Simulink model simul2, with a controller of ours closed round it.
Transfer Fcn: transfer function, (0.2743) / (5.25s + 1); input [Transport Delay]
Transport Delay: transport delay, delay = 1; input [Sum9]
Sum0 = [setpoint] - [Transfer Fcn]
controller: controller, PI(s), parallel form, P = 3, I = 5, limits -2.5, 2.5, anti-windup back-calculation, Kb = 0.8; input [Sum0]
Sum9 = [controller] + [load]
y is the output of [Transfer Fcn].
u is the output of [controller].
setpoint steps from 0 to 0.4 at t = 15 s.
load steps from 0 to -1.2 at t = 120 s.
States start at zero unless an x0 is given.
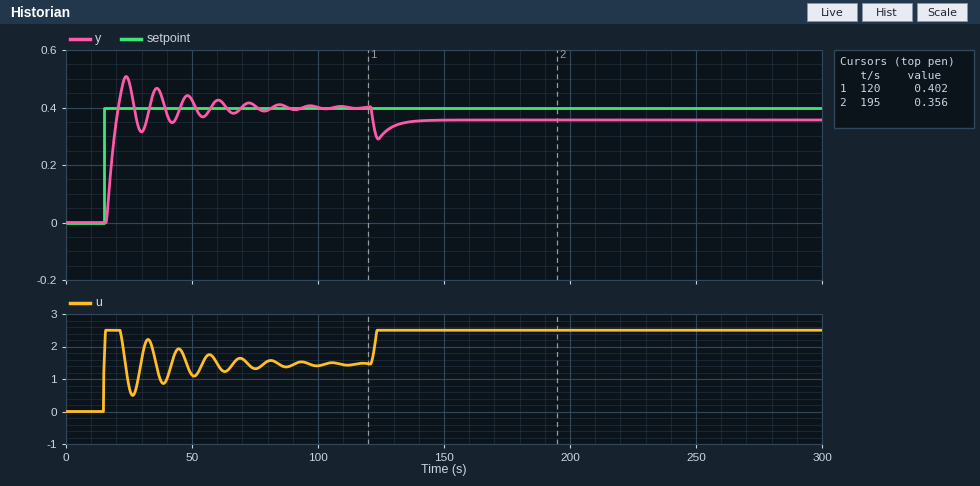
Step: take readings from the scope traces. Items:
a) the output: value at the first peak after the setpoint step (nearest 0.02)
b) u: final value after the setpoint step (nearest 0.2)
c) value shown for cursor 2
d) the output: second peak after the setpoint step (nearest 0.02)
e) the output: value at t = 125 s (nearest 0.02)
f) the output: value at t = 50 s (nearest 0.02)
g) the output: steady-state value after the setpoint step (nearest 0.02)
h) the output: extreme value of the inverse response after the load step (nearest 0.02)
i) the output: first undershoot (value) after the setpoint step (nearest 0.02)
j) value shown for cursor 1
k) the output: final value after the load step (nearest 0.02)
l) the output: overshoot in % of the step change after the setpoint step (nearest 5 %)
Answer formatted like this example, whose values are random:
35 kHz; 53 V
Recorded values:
0.50; 1.4; 0.356; 0.46; 0.30; 0.42; 0.40; 0.40; 0.32; 0.402; 0.36; 25 %
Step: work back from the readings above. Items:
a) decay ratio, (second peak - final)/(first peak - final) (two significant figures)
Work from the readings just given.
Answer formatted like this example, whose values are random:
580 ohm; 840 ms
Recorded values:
0.60
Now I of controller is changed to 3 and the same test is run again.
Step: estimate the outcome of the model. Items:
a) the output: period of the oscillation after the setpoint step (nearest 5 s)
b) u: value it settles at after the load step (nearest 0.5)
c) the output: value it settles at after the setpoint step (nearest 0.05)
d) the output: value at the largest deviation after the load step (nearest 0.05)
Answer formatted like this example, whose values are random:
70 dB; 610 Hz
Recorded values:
15 s; 2.5; 0.40; 0.30
